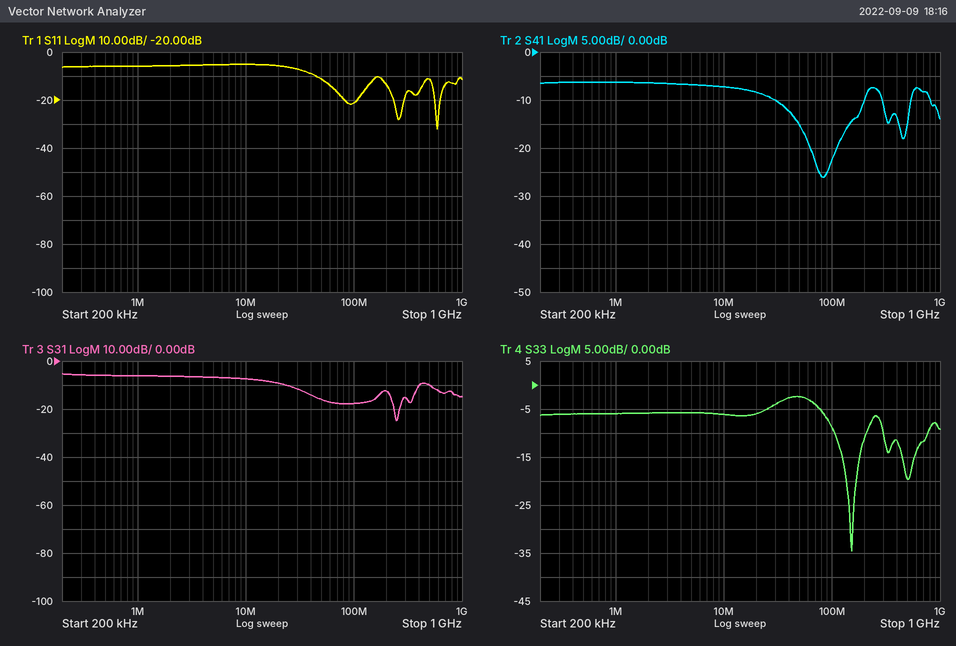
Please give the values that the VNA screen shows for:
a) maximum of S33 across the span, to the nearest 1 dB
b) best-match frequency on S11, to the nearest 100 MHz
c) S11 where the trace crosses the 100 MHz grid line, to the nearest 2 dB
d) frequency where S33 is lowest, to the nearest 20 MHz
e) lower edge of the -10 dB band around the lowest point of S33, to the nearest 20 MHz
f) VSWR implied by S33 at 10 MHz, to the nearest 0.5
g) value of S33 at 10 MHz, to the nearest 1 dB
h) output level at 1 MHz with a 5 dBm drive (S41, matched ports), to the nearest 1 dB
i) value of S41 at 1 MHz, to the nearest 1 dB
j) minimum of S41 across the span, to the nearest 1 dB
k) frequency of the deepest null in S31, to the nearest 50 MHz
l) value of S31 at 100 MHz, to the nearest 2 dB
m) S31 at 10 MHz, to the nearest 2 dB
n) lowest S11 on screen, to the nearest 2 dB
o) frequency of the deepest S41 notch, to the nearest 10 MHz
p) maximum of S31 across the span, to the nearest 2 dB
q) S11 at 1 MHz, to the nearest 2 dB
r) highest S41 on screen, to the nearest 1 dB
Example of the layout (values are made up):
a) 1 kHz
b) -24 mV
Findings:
a) -2 dB
b) 600 MHz
c) -22 dB
d) 160 MHz
e) 100 MHz
f) 3.0
g) -6 dB
h) -1 dBm
i) -6 dB
j) -26 dB
k) 250 MHz
l) -18 dB
m) -8 dB
n) -32 dB
o) 80 MHz
p) -6 dB
q) -6 dB
r) -6 dB
